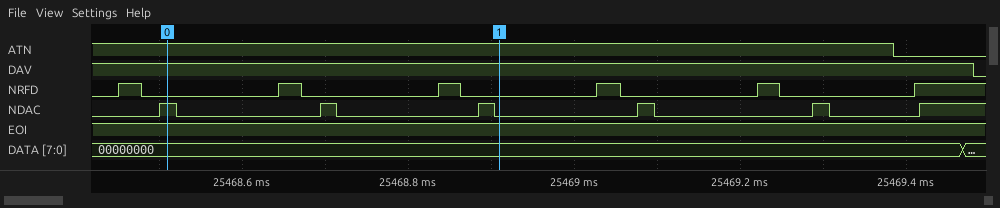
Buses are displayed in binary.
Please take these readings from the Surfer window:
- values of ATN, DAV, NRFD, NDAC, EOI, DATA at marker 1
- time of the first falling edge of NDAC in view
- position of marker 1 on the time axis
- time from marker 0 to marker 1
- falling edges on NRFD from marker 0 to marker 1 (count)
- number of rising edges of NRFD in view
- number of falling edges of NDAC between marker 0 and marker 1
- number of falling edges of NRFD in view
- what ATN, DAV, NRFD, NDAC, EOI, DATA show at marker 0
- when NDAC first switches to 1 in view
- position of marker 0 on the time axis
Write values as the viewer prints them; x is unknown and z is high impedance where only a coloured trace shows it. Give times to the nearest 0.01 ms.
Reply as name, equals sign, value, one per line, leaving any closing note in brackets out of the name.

values of ATN, DAV, NRFD, NDAC, EOI, DATA at marker 1 = ATN=1, DAV=1, NRFD=0, NDAC=0, EOI=1, DATA=00000000
time of the first falling edge of NDAC in view = 25468.52 ms
position of marker 1 on the time axis = 25468.91 ms
time from marker 0 to marker 1 = 0.4 ms
falling edges on NRFD from marker 0 to marker 1 = 2
number of rising edges of NRFD in view = 6
number of falling edges of NDAC between marker 0 and marker 1 = 3
number of falling edges of NRFD in view = 5
what ATN, DAV, NRFD, NDAC, EOI, DATA show at marker 0 = ATN=1, DAV=1, NRFD=0, NDAC=1, EOI=1, DATA=00000000
when NDAC first switches to 1 in view = 25468.5 ms
position of marker 0 on the time axis = 25468.51 ms
